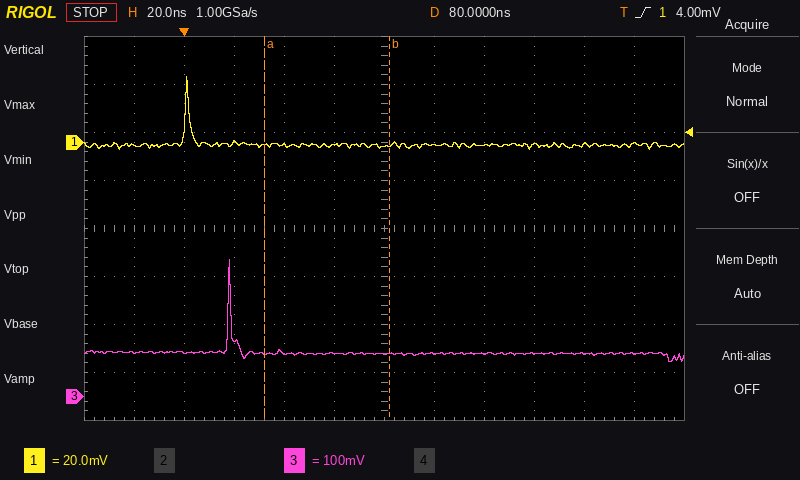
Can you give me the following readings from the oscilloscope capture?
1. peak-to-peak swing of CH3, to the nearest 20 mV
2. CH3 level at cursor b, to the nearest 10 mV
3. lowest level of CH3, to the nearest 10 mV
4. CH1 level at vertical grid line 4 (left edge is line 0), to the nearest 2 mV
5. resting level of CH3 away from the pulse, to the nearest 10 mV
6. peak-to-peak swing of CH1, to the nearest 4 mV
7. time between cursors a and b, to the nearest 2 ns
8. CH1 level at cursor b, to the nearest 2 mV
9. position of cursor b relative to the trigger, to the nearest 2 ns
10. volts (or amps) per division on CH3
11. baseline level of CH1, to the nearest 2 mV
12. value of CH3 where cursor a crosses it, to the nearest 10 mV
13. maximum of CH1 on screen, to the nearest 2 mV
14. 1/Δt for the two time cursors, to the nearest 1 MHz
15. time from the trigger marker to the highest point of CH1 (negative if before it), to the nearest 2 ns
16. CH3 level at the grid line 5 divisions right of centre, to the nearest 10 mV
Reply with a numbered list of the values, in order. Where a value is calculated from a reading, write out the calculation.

1. 220 mV
2. 90 mV
3. 70 mV
4. -2 mV
5. 90 mV
6. 32 mV
7. 50 ns
8. -2 mV
9. +82 ns
10. 100 mV
11. -2 mV
12. 90 mV
13. 28 mV
14. 1 / 50 ns ≈ 20 MHz
15. +2 ns
16. 90 mV
